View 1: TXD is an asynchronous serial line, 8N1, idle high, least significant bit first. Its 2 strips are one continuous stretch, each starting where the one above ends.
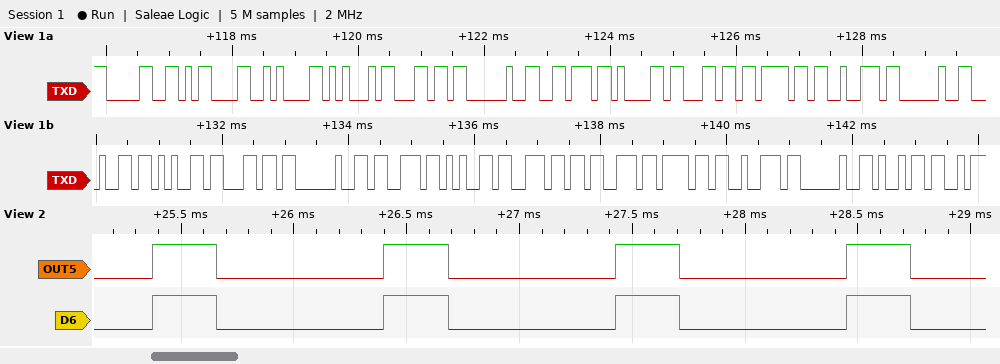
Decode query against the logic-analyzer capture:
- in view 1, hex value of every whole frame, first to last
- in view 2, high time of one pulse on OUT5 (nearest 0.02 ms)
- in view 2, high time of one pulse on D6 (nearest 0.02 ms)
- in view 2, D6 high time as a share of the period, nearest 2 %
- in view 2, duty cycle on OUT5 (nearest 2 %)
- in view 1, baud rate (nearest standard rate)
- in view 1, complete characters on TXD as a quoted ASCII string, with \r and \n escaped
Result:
30 0D 0A 45 6C 20 76 61 6C 6F 72 20 64 65 6C 20 73 65 6E 73 6F 72 20 69
0.28 ms
0.28 ms
28 %
28 %
9600 baud
"0\r\nEl valor del sensor i"
